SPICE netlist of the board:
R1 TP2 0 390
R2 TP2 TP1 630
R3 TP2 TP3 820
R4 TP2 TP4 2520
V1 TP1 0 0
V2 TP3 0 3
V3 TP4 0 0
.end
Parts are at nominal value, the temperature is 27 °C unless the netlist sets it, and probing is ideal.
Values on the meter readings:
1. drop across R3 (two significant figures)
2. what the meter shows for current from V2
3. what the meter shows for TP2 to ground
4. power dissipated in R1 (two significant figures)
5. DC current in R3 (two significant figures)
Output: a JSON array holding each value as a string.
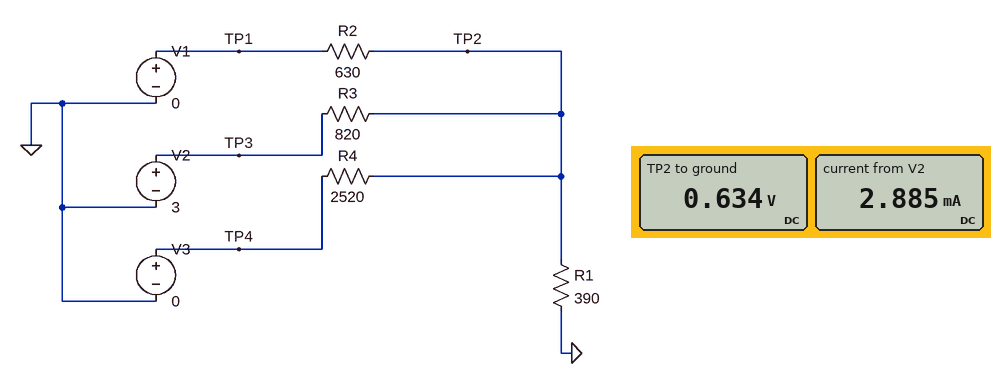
["2.4 V", "2.885 mA", "0.634 V", "1.0 mW", "2.9 mA"]
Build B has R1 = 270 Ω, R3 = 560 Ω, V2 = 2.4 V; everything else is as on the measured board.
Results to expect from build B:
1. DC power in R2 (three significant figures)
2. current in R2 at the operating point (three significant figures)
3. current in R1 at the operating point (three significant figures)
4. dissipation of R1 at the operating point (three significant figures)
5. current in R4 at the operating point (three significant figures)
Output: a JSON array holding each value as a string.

["522 µW", "910 µA", "2.12 mA", "1.22 mW", "228 µA"]
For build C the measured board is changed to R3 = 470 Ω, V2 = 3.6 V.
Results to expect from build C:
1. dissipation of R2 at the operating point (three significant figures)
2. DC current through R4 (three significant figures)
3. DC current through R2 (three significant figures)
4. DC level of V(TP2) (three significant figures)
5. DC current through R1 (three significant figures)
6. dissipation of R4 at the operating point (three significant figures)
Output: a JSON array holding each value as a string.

["2.09 mW", "455 µA", "1.82 mA", "1.15 V", "2.94 mA", "522 µW"]
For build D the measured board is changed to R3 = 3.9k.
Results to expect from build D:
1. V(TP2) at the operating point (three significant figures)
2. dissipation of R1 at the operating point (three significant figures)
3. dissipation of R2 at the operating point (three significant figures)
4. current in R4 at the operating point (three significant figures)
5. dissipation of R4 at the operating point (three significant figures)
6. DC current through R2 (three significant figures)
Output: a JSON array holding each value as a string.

["160 mV", "65.7 µW", "40.7 µW", "63.5 µA", "10.2 µW", "254 µA"]
